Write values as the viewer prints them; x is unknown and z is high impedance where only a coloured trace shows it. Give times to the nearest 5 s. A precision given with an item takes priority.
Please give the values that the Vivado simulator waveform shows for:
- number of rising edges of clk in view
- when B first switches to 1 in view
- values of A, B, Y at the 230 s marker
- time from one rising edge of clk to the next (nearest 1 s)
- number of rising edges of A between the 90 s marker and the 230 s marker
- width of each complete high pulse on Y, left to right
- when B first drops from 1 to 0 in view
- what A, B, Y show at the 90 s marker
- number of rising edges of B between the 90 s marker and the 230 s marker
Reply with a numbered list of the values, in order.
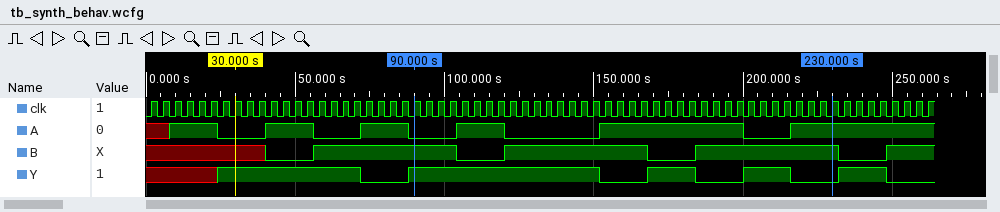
1. 66
2. 55 s
3. A=1, B=1, Y=0
4. 4 s
5. 3
6. 65 s, 15 s, 15 s, 15 s
7. 105 s
8. A=0, B=1, Y=1
9. 2
